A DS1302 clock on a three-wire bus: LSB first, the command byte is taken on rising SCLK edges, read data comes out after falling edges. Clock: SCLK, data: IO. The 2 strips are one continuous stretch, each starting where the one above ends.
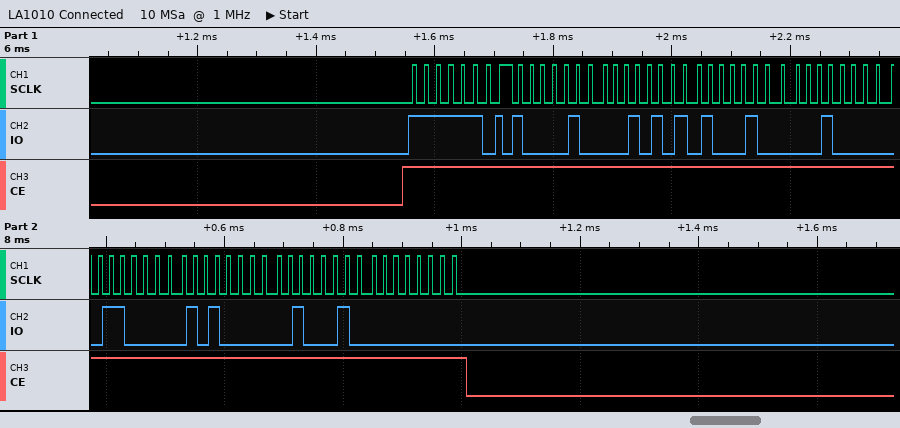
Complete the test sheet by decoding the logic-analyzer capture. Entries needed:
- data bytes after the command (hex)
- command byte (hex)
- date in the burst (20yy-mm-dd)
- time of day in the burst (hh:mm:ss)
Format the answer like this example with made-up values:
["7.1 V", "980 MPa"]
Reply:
["21 54 11 04 06 05 22 00", "0xBF", "2022-06-04", "11:54:21"]
